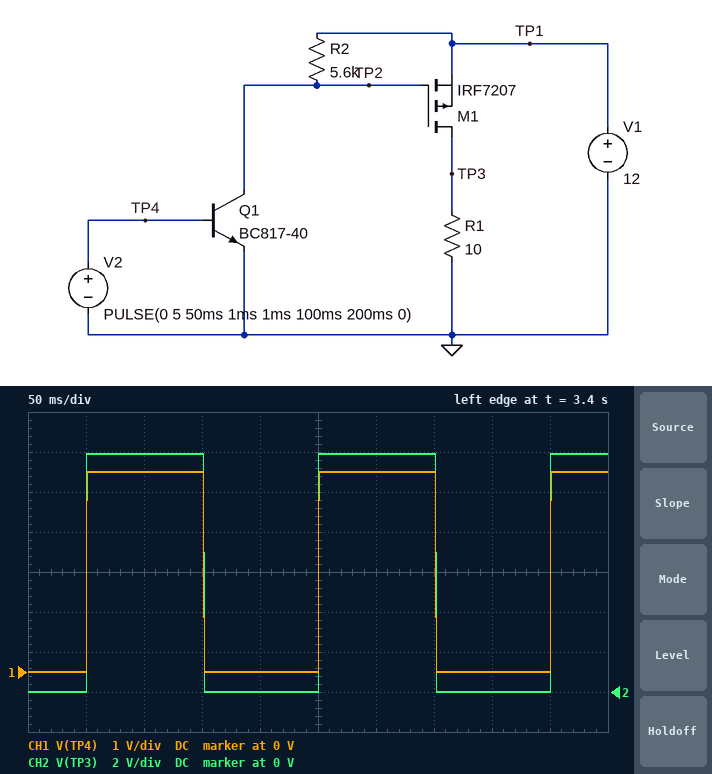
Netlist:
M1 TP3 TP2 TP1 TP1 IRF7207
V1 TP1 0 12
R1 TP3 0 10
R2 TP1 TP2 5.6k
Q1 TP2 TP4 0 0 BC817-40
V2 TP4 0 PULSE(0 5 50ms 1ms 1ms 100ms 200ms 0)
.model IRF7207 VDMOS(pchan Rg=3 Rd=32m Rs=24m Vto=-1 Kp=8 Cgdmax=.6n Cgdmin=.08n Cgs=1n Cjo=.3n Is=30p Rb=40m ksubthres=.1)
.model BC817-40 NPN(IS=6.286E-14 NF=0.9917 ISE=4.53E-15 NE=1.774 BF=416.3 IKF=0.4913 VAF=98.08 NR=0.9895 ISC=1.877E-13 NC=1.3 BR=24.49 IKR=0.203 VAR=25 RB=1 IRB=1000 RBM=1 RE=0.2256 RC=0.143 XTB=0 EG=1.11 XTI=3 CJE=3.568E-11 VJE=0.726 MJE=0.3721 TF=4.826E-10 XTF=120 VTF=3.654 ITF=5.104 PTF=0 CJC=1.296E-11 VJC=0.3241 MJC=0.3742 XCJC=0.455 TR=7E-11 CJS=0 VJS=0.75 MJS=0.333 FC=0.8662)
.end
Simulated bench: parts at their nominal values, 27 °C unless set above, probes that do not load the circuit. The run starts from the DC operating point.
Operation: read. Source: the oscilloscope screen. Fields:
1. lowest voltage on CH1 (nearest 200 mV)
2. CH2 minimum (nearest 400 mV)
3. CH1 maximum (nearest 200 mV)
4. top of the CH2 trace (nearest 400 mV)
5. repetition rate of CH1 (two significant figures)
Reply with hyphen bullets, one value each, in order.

- 0 V
- 0 V
- 5.0 V
- 12.0 V
- 5.0 Hz
